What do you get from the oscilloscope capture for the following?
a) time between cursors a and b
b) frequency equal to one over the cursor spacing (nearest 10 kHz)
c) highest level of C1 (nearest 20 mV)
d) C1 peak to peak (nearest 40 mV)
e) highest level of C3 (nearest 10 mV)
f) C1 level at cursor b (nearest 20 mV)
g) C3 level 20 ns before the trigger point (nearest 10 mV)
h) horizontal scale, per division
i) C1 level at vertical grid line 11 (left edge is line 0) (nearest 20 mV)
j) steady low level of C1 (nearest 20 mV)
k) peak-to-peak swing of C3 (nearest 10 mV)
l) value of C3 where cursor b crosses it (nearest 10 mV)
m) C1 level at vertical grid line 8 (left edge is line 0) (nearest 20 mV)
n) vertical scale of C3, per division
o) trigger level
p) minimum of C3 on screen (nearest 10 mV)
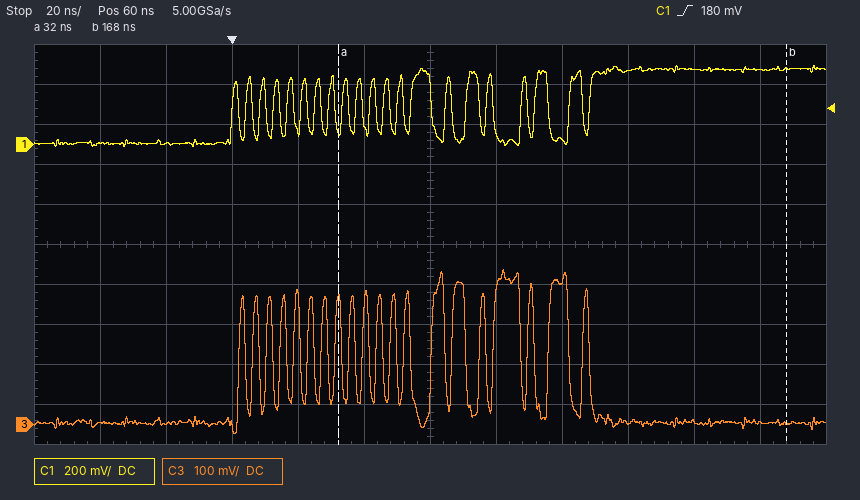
136 ns
7.35 MHz
400 mV
400 mV
390 mV
380 mV
0 mV
20 ns
380 mV
0 mV
410 mV
0 mV
20 mV
100 mV
180 mV
-20 mV
